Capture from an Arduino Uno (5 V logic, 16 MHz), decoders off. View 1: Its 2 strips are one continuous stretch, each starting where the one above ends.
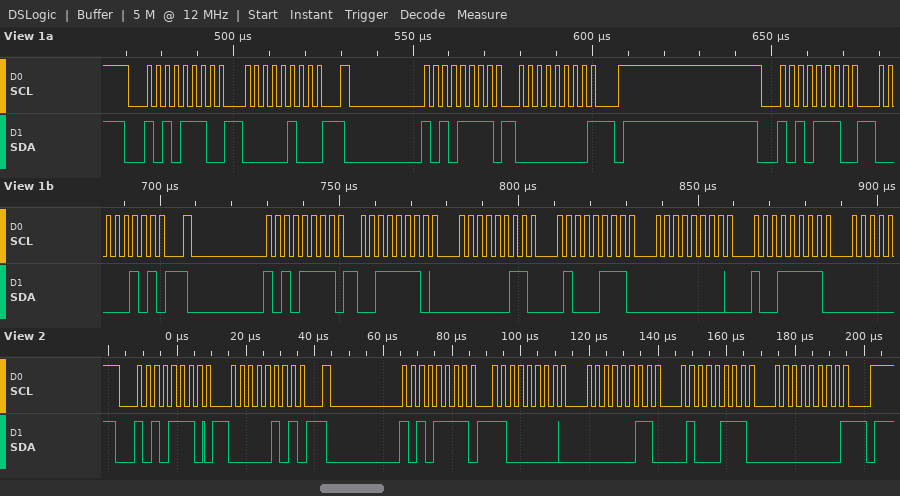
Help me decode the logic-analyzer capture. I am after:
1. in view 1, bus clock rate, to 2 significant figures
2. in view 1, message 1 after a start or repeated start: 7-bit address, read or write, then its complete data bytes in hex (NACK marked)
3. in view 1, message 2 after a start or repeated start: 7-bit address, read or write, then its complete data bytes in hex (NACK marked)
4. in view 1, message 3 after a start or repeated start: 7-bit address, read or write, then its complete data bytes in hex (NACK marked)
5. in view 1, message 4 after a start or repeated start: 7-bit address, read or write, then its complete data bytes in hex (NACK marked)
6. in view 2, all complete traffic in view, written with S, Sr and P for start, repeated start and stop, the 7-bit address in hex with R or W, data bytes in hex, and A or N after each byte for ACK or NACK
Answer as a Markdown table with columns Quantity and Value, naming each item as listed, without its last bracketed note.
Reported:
| Quantity | Value |
|---|---|
| in view 1, bus clock rate, to 2 significant figures | 400 kHz |
| in view 1, message 1 after a start or repeated start: 7-bit address, read or write, then its complete data bytes in hex | 0x57 write: 04 |
| in view 1, message 2 after a start or repeated start: 7-bit address, read or write, then its complete data bytes in hex | 0x57 read: 00 NACK |
| in view 1, message 3 after a start or repeated start: 7-bit address, read or write, then its complete data bytes in hex | 0x57 write: 05 |
| in view 1, message 4 after a start or repeated start: 7-bit address, read or write, then its complete data bytes in hex | 0x57 read: 3E 03 47 00 9F |
| in view 2, all complete traffic in view, written with S, Sr and P for start, repeated start and stop, the 7-bit address in hex with R or W, data bytes in hex, and A or N after each byte for ACK or NACK | S 57W A 05 A Sr 57R A C0 A 03 A 47 A 00 N P |
